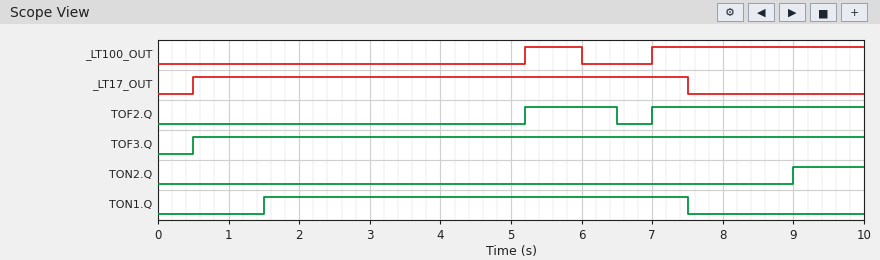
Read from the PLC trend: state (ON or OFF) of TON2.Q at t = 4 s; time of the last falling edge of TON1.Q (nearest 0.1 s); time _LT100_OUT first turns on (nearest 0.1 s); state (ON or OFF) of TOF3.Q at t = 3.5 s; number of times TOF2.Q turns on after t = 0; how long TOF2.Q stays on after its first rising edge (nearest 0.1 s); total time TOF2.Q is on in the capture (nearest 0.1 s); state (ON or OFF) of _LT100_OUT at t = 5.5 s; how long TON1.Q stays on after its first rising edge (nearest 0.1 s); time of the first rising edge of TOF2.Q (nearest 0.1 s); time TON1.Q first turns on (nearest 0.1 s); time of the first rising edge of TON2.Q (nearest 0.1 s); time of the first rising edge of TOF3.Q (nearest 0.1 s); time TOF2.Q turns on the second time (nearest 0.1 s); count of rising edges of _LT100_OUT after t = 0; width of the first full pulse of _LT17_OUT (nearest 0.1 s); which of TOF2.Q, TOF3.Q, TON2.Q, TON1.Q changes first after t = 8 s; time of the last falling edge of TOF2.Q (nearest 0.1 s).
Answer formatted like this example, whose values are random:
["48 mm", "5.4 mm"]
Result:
["OFF", "7.5 s", "5.2 s", "ON", "2", "1.3 s", "4.3 s", "ON", "6.0 s", "5.2 s", "1.5 s", "9.0 s", "0.5 s", "7.0 s", "2", "7.0 s", "TON2.Q", "6.5 s"]
